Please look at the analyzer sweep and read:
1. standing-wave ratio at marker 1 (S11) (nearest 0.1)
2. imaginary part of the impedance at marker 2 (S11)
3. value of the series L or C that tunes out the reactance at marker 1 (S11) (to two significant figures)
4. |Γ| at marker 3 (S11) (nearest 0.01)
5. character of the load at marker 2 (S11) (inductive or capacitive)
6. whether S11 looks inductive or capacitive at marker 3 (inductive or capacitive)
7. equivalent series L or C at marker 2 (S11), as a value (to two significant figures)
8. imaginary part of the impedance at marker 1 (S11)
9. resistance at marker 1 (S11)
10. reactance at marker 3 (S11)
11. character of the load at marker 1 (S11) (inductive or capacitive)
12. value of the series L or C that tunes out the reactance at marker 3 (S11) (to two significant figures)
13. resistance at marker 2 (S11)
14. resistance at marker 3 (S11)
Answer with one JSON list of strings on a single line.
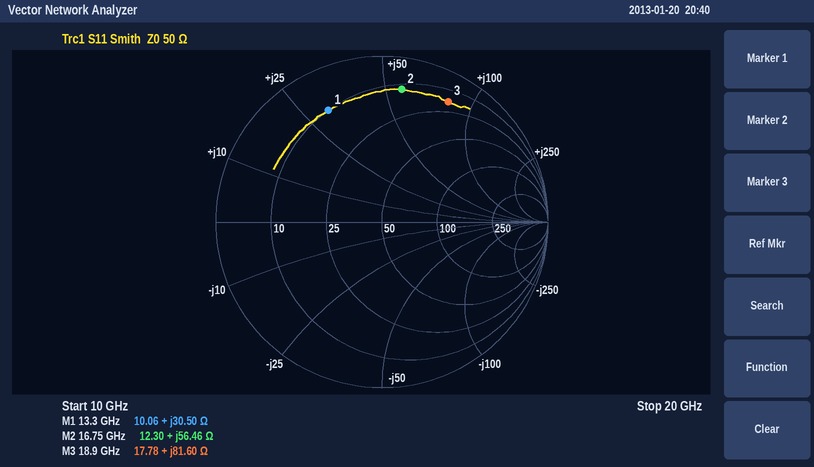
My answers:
["6.9", "+56.46 Ω", "390 fF", "0.83", "inductive", "inductive", "540 pH", "+30.50 Ω", "10.06 Ω", "+81.60 Ω", "inductive", "100 fF", "12.30 Ω", "17.78 Ω"]
